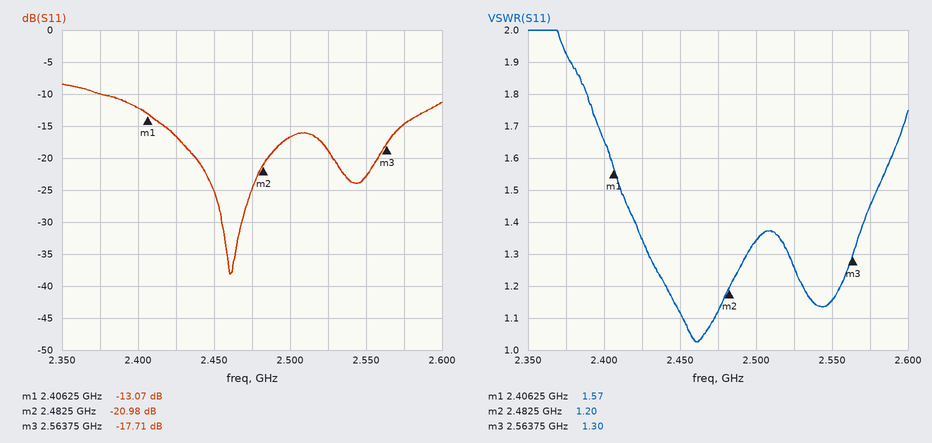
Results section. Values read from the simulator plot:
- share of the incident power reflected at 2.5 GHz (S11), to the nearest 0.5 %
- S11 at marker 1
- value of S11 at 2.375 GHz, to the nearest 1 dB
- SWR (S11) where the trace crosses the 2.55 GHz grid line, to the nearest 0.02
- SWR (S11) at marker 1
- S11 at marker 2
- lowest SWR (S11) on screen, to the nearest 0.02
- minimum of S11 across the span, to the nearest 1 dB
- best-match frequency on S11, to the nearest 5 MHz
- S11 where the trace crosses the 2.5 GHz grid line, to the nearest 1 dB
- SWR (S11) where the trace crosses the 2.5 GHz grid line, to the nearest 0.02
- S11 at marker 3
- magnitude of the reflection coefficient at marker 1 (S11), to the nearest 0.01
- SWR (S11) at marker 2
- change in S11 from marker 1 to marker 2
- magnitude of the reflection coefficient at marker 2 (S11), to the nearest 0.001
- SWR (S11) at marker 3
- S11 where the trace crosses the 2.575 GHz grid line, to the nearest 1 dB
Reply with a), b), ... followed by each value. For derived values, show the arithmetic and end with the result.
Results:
a) 10^(-17/10) ≈ 2.0 %
b) -13.07 dB
c) -10 dB
d) 1.16
e) 1.57
f) -20.98 dB
g) 1.02
h) -38 dB
i) 2.460 GHz
j) -17 dB
k) 1.34
l) -17.71 dB
m) 10^(-13.07/20) ≈ 0.22
n) 1.20
o) -20.98 − (-13.07) = -7.91 dB
p) 10^(-20.98/20) ≈ 0.089
q) 1.30
r) -15 dB
